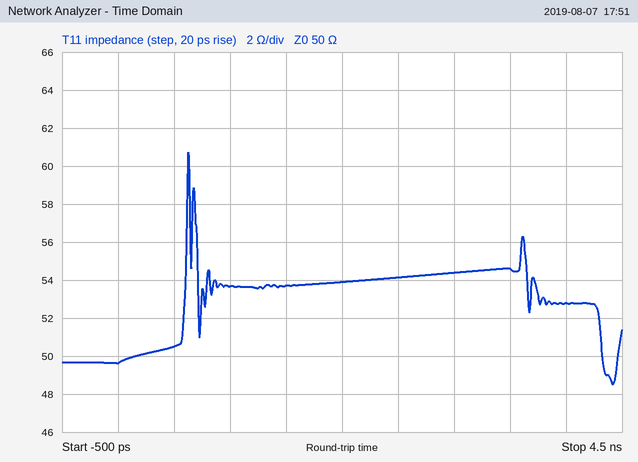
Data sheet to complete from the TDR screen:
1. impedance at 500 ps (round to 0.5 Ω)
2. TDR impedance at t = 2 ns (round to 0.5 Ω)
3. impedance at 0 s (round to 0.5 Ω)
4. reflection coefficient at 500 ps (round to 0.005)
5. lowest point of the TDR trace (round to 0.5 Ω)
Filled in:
50.5 Ω
54.0 Ω
49.5 Ω
+0.005
48.5 Ω
